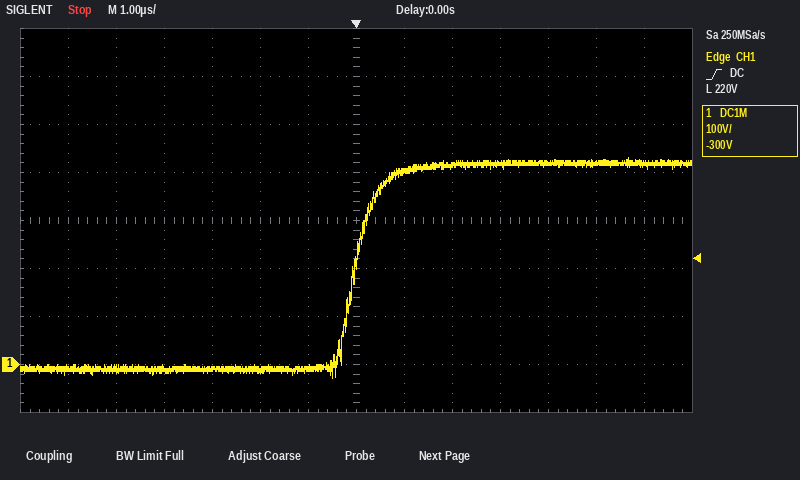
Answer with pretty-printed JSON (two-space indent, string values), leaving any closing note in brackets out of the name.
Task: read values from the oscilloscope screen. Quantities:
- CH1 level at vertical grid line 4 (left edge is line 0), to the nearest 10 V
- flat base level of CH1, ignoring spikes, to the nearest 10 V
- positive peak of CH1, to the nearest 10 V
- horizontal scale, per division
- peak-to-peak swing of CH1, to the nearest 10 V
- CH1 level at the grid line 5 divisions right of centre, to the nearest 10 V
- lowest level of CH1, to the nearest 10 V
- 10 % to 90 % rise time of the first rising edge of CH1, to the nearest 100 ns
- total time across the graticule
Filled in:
{
  "CH1 level at vertical grid line 4 (left edge is line 0), to the nearest 10 V": "-10 V",
  "flat base level of CH1, ignoring spikes, to the nearest 10 V": "-10 V",
  "positive peak of CH1, to the nearest 10 V": "430 V",
  "horizontal scale, per division": "1 µs",
  "peak-to-peak swing of CH1, to the nearest 10 V": "460 V",
  "CH1 level at the grid line 5 divisions right of centre, to the nearest 10 V": "420 V",
  "lowest level of CH1, to the nearest 10 V": "-30 V",
  "10 % to 90 % rise time of the first rising edge of CH1, to the nearest 100 ns": "900 ns",
  "total time across the graticule": "14 µs"
}
